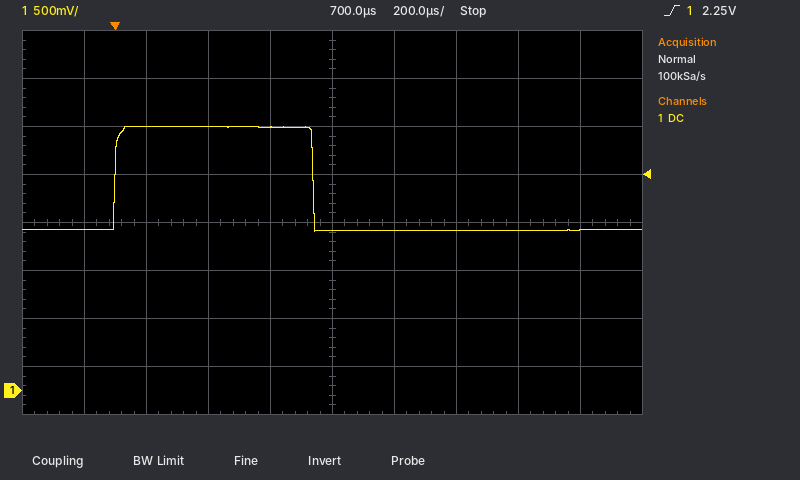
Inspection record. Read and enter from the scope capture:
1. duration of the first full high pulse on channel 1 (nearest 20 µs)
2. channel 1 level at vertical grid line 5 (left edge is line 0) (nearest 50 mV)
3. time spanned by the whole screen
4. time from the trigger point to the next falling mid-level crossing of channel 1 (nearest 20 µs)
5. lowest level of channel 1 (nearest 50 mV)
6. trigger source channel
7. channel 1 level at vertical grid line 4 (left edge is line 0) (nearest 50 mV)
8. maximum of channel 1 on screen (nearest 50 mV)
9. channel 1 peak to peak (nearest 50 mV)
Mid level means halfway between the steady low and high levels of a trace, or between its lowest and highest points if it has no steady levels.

640 µs
1.65 V
2 ms
640 µs
1.65 V
channel 1
2.75 V
2.75 V
1.10 V
